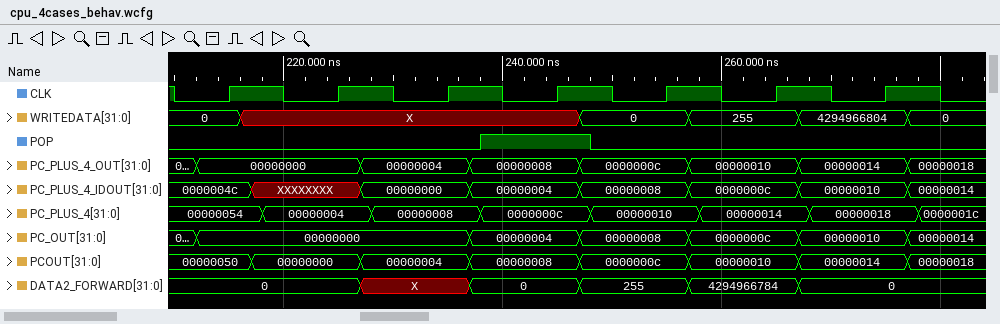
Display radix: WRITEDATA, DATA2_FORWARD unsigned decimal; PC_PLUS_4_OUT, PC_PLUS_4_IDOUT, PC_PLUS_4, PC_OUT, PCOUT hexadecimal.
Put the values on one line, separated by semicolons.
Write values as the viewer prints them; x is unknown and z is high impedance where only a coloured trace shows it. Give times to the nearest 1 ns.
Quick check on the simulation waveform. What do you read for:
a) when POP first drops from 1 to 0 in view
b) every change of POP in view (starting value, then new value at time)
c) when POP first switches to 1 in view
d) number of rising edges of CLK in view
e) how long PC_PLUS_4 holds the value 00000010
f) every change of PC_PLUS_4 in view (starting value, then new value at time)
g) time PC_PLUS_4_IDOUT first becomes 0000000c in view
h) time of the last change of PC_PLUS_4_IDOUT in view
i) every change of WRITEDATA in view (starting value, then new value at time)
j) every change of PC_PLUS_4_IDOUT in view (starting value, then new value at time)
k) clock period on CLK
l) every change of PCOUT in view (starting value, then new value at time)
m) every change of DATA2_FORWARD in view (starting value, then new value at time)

248 ns; 0, 1 at 238 ns, 0 at 248 ns; 238 ns; 7; 10 ns; 00000054, 00000004 at 218 ns, 00000008 at 228 ns, 0000000c at 238 ns, 00000010 at 248 ns, 00000014 at 258 ns, 00000018 at 268 ns, 0000001c at 278 ns; 257 ns; 277 ns; 0, X at 216 ns, 0 at 247 ns, 255 at 257 ns, 4294966804 at 267 ns, 0 at 277 ns; 0000004c, XXXXXXXX at 217 ns, 00000000 at 227 ns, 00000004 at 237 ns, 00000008 at 247 ns, 0000000c at 257 ns, 00000010 at 267 ns, 00000014 at 277 ns; 10 ns; 00000050, 00000000 at 217 ns, 00000004 at 227 ns, 00000008 at 237 ns, 0000000c at 247 ns, 00000010 at 257 ns, 00000014 at 267 ns, 00000018 at 277 ns; 0, X at 227 ns, 0 at 237 ns, 255 at 247 ns, 4294966784 at 257 ns, 0 at 267 ns
